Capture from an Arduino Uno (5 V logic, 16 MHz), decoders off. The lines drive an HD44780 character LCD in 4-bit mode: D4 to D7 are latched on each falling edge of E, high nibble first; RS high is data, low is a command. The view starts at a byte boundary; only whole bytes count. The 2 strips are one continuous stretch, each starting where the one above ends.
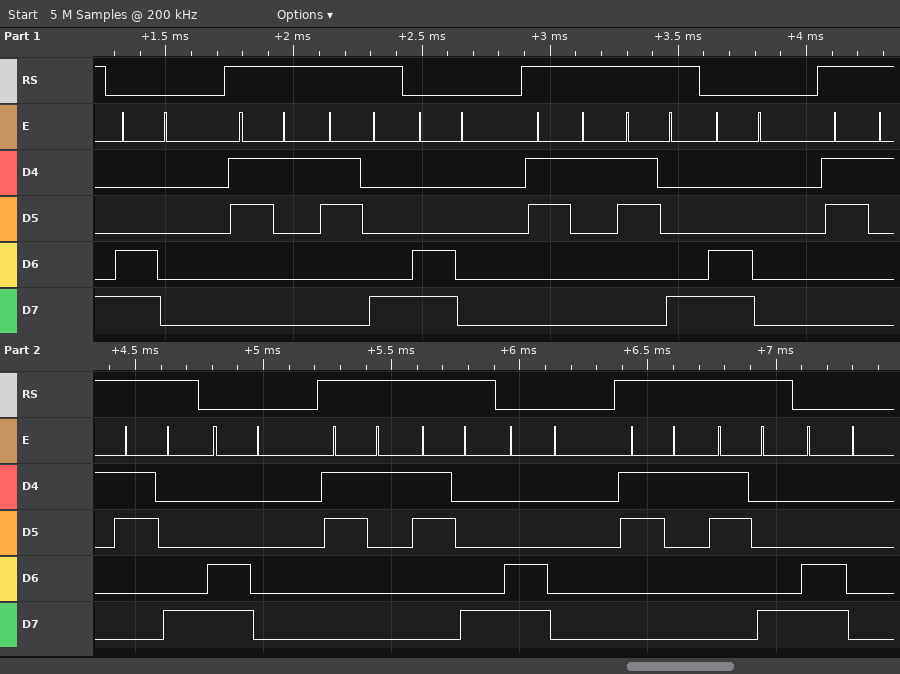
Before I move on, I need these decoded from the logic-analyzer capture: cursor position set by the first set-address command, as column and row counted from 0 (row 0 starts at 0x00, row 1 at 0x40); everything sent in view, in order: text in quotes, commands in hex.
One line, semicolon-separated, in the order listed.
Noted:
column 0, row 1; 0xC0 "18" 0xC0 "18" 0xC0 "18" 0xC0 "18" 0xC0 "18" 0xC0
